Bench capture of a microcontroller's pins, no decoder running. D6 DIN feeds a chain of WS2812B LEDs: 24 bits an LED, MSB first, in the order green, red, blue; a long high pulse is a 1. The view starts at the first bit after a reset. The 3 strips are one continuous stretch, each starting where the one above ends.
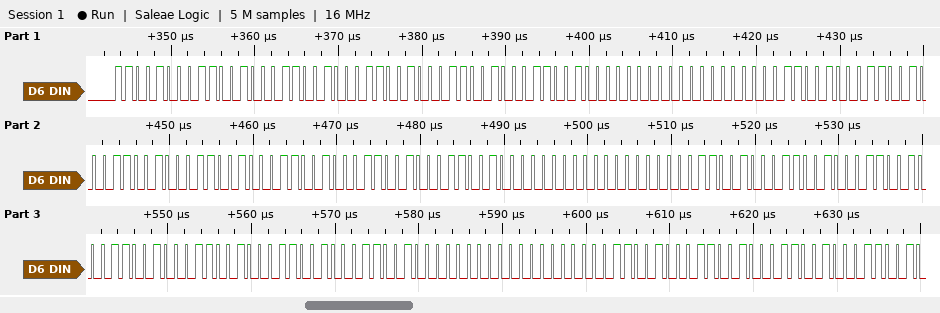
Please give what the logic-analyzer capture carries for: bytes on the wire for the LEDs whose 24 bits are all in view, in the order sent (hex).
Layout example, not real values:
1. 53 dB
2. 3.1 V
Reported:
1. C8 C8 C8 C8 C8 C8 00 00 C8 C8 C8 C8 C8 C8 C8 00 00 C8 C8 C8 C8 C8 C8 C8 00 00 C8
